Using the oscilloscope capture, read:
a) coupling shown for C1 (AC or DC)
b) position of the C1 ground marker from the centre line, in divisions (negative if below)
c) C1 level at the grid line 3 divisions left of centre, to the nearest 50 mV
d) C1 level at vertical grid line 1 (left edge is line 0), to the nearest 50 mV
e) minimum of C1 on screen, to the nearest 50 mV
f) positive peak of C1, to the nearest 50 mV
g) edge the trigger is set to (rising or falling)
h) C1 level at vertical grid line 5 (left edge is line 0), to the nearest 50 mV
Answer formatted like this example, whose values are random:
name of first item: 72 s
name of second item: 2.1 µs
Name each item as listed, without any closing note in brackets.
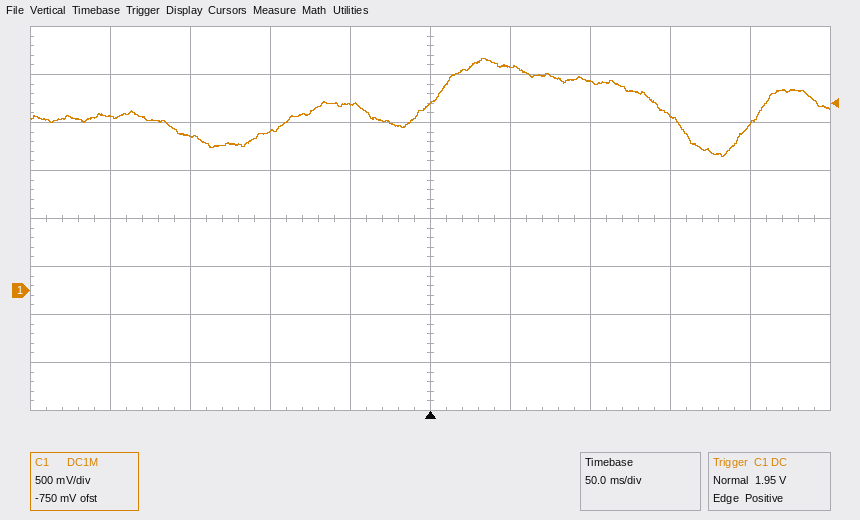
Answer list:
coupling shown for C1: DC
position of the C1 ground marker from the centre line, in divisions: -1.5 div
C1 level at the grid line 3 divisions left of centre, to the nearest 50 mV: 1.60 V
C1 level at vertical grid line 1 (left edge is line 0), to the nearest 50 mV: 1.80 V
minimum of C1 on screen, to the nearest 50 mV: 1.40 V
positive peak of C1, to the nearest 50 mV: 2.40 V
edge the trigger is set to: rising
C1 level at vertical grid line 5 (left edge is line 0), to the nearest 50 mV: 1.95 V
